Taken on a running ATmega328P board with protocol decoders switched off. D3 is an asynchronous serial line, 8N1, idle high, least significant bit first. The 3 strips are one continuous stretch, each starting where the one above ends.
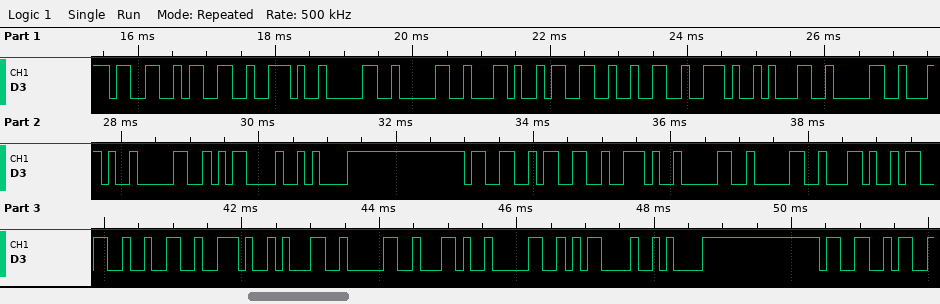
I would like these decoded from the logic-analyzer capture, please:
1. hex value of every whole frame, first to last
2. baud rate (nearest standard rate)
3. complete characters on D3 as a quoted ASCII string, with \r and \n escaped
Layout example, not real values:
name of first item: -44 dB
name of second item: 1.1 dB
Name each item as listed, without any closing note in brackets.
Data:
hex value of every whole frame, first to last: 0x33 0x33 0x2E 0x30 0x30 0x2C 0x33 0x32 0x2E 0x31 0x30 0x2C 0x30 0x0D 0x0A 0x33 0x33 0x2E 0x30 0x30 0x2C 0x33 0x32 0x2E 0x31 0x30 0x2C 0x30 0x0D 0x0A 0x33
baud rate: 9600 baud
complete characters on D3 as a quoted ASCII string, with \r and \n escaped: "33.00,32.10,0\r\n33.00,32.10,0\r\n3"
